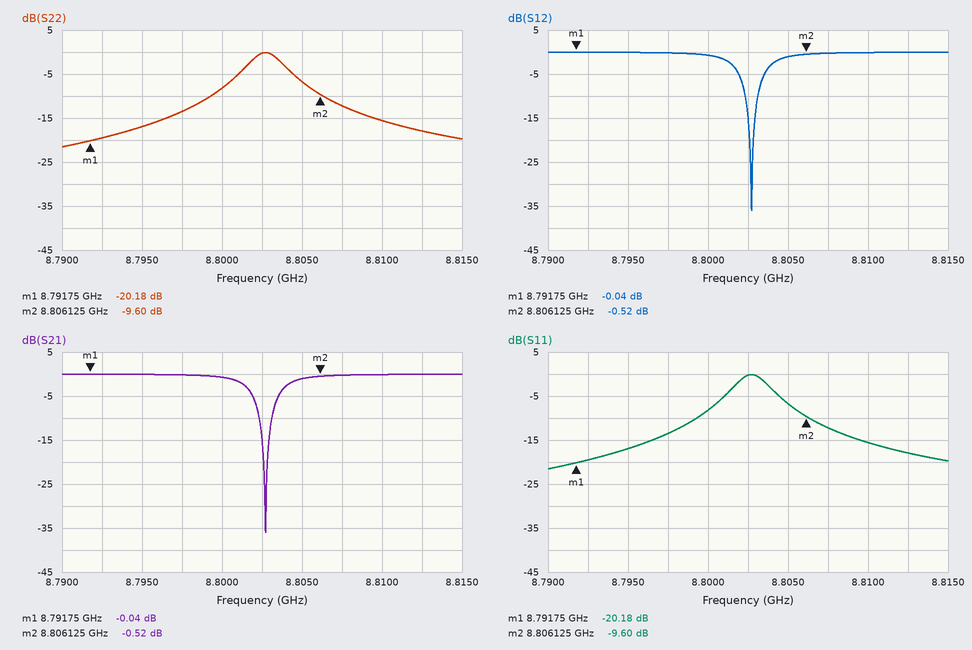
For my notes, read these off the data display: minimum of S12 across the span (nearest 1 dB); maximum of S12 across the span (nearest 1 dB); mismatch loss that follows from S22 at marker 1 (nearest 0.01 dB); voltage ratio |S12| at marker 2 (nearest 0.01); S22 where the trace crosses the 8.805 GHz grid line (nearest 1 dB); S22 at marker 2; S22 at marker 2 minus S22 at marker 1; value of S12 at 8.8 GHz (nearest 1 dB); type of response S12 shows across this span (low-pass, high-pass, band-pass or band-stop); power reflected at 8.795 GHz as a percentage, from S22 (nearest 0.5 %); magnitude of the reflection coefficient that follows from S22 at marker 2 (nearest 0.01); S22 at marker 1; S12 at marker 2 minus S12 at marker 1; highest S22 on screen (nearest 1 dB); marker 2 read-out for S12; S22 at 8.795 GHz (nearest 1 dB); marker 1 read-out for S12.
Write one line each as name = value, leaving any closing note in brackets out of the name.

minimum of S12 across the span = -36 dB
maximum of S12 across the span = 0 dB
mismatch loss that follows from S22 at marker 1 = 0.04 dB
voltage ratio |S12| at marker 2 = 0.94
S22 where the trace crosses the 8.805 GHz grid line = -7 dB
S22 at marker 2 = -9.60 dB
S22 at marker 2 minus S22 at marker 1 = 10.58 dB
value of S12 at 8.8 GHz = -1 dB
type of response S12 shows across this span = band-stop
power reflected at 8.795 GHz as a percentage, from S22 = 2.0 %
magnitude of the reflection coefficient that follows from S22 at marker 2 = 0.33
S22 at marker 1 = -20.18 dB
S12 at marker 2 minus S12 at marker 1 = -0.48 dB
highest S22 on screen = 0 dB
marker 2 read-out for S12 = -0.52 dB
S22 at 8.795 GHz = -17 dB
marker 1 read-out for S12 = -0.04 dB
